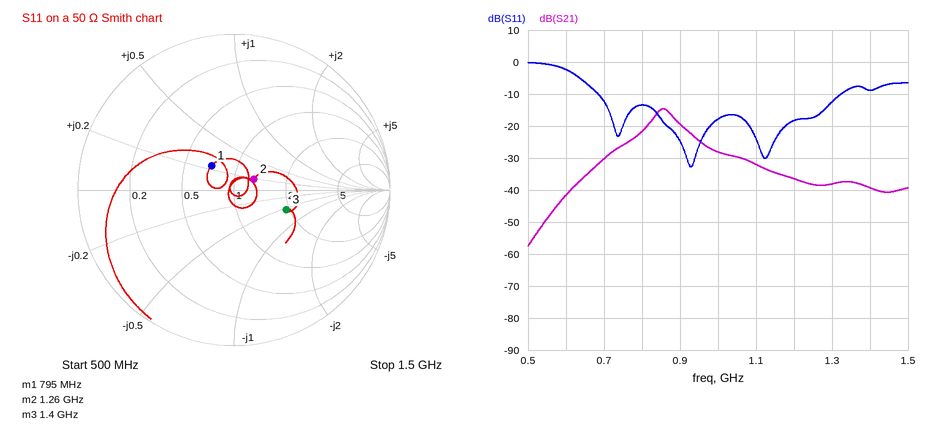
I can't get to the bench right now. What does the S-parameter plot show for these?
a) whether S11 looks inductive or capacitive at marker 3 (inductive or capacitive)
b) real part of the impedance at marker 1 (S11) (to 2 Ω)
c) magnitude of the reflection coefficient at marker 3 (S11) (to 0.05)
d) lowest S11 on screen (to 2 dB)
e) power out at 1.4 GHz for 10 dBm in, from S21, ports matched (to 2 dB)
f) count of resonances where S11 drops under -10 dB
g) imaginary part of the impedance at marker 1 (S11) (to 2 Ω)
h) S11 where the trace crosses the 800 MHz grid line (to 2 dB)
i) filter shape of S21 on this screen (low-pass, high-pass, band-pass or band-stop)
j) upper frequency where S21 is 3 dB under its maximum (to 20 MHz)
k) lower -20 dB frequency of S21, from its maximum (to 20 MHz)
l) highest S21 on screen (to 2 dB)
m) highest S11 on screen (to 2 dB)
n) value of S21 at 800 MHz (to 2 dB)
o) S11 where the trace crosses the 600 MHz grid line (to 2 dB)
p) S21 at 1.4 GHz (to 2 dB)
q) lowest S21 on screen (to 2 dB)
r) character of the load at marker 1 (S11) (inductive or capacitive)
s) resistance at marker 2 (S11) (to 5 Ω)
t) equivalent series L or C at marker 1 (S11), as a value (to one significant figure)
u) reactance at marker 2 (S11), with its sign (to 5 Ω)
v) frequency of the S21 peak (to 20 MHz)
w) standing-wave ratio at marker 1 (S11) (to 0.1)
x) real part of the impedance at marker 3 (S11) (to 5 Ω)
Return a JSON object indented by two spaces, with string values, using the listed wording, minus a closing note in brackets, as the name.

{
  "whether S11 looks inductive or capacitive at marker 3": "capacitive",
  "real part of the impedance at marker 1 (S11)": "36 Ω",
  "magnitude of the reflection coefficient at marker 3 (S11)": "0.35",
  "lowest S11 on screen": "-32 dB",
  "power out at 1.4 GHz for 10 dBm in, from S21, ports matched": "-30 dBm",
  "count of resonances where S11 drops under -10 dB": "3",
  "imaginary part of the impedance at marker 1 (S11)": "+12 Ω",
  "S11 where the trace crosses the 800 MHz grid line": "-14 dB",
  "filter shape of S21 on this screen": "band-pass",
  "upper frequency where S21 is 3 dB under its maximum": "880 MHz",
  "lower -20 dB frequency of S21, from its maximum": "660 MHz",
  "highest S21 on screen": "-14 dB",
  "highest S11 on screen": "0 dB",
  "value of S21 at 800 MHz": "-22 dB",
  "S11 where the trace crosses the 600 MHz grid line": "-2 dB",
  "S21 at 1.4 GHz": "-40 dB",
  "lowest S21 on screen": "-58 dB",
  "character of the load at marker 1 (S11)": "inductive",
  "resistance at marker 2 (S11)": "65 Ω",
  "equivalent series L or C at marker 1 (S11), as a value": "2 nH",
  "reactance at marker 2 (S11), with its sign": "+10 Ω",
  "frequency of the S21 peak": "860 MHz",
  "standing-wave ratio at marker 1 (S11)": "1.5",
  "real part of the impedance at marker 3 (S11)": "95 Ω"
}
